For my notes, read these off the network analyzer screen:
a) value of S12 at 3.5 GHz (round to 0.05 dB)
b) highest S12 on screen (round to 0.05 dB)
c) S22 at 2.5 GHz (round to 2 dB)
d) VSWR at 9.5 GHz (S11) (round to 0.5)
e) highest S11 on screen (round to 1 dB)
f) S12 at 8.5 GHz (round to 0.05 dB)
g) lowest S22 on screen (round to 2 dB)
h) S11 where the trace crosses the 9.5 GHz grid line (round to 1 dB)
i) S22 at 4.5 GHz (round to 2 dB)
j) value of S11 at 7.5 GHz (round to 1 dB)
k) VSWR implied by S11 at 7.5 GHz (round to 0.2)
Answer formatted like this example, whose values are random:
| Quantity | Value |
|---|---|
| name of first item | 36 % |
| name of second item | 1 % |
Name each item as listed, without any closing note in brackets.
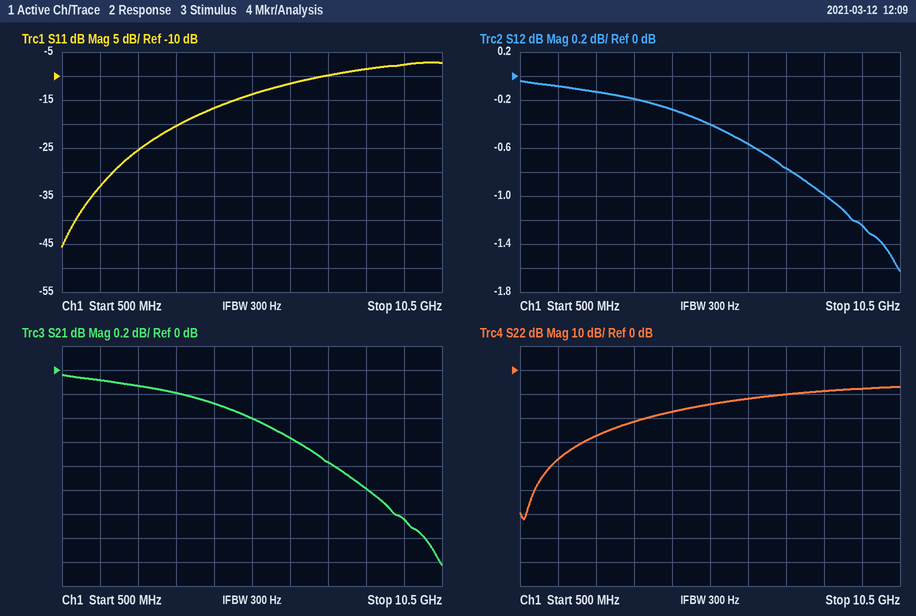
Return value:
| Quantity | Value |
|---|---|
| value of S12 at 3.5 GHz | -0.20 dB |
| highest S12 on screen | -0.05 dB |
| S22 at 2.5 GHz | -28 dB |
| VSWR at 9.5 GHz (S11) | 2.5 |
| highest S11 on screen | -7 dB |
| S12 at 8.5 GHz | -1.00 dB |
| lowest S22 on screen | -62 dB |
| S11 where the trace crosses the 9.5 GHz grid line | -8 dB |
| S22 at 4.5 GHz | -18 dB |
| value of S11 at 7.5 GHz | -10 dB |
| VSWR implied by S11 at 7.5 GHz | 2.0 |
